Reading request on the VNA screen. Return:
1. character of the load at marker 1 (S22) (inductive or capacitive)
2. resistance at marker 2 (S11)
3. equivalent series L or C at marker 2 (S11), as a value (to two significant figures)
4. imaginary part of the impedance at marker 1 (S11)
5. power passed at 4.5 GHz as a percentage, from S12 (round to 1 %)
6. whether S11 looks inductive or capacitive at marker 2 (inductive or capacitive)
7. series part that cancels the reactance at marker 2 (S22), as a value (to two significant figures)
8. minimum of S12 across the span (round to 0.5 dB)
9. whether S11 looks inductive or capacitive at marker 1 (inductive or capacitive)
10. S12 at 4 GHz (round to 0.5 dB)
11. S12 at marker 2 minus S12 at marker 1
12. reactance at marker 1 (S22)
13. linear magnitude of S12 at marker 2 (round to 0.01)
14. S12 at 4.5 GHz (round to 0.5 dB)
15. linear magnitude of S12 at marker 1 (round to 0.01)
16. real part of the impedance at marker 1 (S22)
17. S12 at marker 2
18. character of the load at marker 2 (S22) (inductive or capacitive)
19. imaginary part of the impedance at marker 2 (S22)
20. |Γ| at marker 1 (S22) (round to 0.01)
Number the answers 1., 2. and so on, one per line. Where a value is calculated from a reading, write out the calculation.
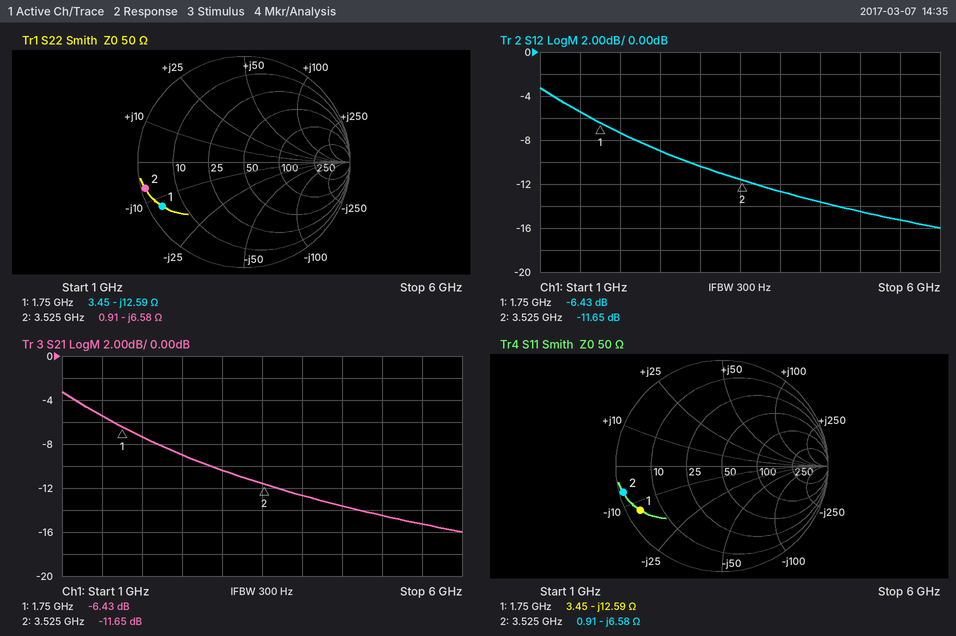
1. capacitive
2. 0.91 Ω
3. C = 1/(2π × 3.525 GHz × 6.58 Ω) ≈ 6.9 pF
4. -12.59 Ω
5. 10^(-13.5/10) ≈ 4 %
6. capacitive
7. L = 6.58 Ω/(2π × 3.525 GHz) ≈ 297 pH, so 300 pH to two significant figures
8. -16.0 dB
9. capacitive
10. -12.5 dB
11. -11.65 − (-6.43) = -5.22 dB
12. -12.59 Ω
13. 10^(-11.65/20) ≈ 0.26
14. -13.5 dB
15. 10^(-6.43/20) ≈ 0.48
16. 3.45 Ω
17. -11.65 dB
18. capacitive
19. -6.58 Ω
20. 0.88
